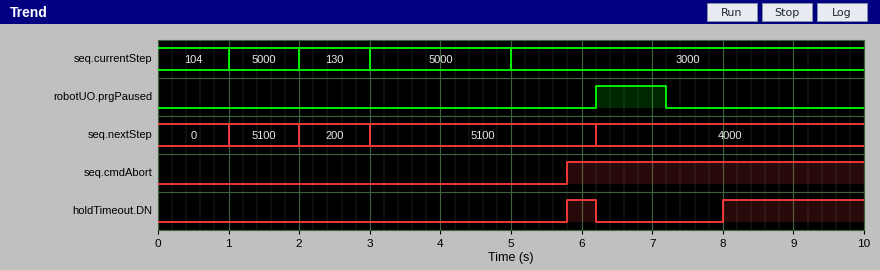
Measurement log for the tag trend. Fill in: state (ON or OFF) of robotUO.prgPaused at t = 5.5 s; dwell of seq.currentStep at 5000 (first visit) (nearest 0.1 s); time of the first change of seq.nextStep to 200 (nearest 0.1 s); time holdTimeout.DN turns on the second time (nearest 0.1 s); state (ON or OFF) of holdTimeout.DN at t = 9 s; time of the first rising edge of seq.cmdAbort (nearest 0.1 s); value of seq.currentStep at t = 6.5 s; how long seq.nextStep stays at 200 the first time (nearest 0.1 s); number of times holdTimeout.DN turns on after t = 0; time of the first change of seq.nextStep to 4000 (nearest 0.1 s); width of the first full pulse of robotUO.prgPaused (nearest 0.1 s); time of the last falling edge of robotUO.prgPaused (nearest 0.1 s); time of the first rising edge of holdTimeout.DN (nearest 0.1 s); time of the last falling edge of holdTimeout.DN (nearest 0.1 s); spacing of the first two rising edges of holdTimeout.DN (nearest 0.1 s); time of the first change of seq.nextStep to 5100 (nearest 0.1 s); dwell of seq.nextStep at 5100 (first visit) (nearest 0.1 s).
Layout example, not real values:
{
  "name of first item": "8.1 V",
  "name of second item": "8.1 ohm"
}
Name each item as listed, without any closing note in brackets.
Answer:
{
  "state (ON or OFF) of robotUO.prgPaused at t = 5.5 s": "OFF",
  "dwell of seq.currentStep at 5000 (first visit)": "1.0 s",
  "time of the first change of seq.nextStep to 200": "2.0 s",
  "time holdTimeout.DN turns on the second time": "8.0 s",
  "state (ON or OFF) of holdTimeout.DN at t = 9 s": "ON",
  "time of the first rising edge of seq.cmdAbort": "5.8 s",
  "value of seq.currentStep at t = 6.5 s": "3000",
  "how long seq.nextStep stays at 200 the first time": "1.0 s",
  "number of times holdTimeout.DN turns on after t = 0": "2",
  "time of the first change of seq.nextStep to 4000": "6.2 s",
  "width of the first full pulse of robotUO.prgPaused": "1.0 s",
  "time of the last falling edge of robotUO.prgPaused": "7.2 s",
  "time of the first rising edge of holdTimeout.DN": "5.8 s",
  "time of the last falling edge of holdTimeout.DN": "6.2 s",
  "spacing of the first two rising edges of holdTimeout.DN": "2.2 s",
  "time of the first change of seq.nextStep to 5100": "1.0 s",
  "dwell of seq.nextStep at 5100 (first visit)": "1.0 s"
}
